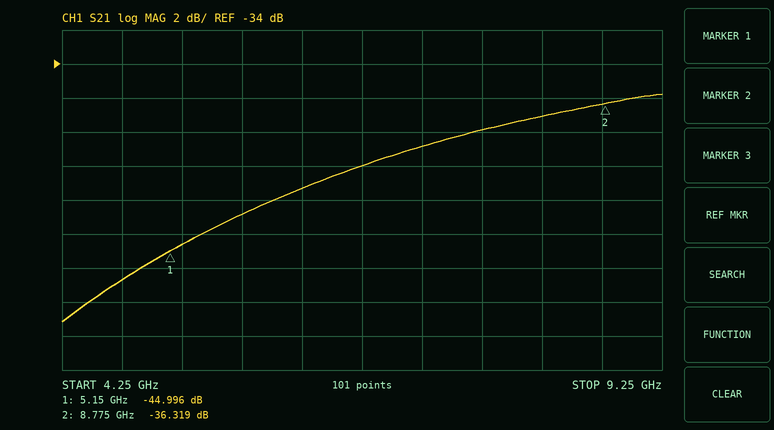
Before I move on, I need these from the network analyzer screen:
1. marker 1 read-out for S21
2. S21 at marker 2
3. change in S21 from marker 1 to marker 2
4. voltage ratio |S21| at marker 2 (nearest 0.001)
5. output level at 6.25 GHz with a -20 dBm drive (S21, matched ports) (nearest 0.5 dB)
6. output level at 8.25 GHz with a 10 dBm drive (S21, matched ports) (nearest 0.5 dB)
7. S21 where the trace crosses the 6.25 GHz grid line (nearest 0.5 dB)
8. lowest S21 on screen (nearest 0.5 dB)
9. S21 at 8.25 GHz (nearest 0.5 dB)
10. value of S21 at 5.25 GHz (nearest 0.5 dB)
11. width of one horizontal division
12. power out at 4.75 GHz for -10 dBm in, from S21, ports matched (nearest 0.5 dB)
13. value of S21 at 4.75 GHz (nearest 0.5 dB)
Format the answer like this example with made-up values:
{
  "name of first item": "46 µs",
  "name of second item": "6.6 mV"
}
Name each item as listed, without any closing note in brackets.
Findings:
{
  "marker 1 read-out for S21": "-44.996 dB",
  "S21 at marker 2": "-36.319 dB",
  "change in S21 from marker 1 to marker 2": "8.677 dB",
  "voltage ratio |S21| at marker 2": "0.015",
  "output level at 6.25 GHz with a -20 dBm drive (S21, matched ports)": "-61.5 dBm",
  "output level at 8.25 GHz with a 10 dBm drive (S21, matched ports)": "-27.0 dBm",
  "S21 where the trace crosses the 6.25 GHz grid line": "-41.5 dB",
  "lowest S21 on screen": "-49.0 dB",
  "S21 at 8.25 GHz": "-37.0 dB",
  "value of S21 at 5.25 GHz": "-44.5 dB",
  "width of one horizontal division": "500 MHz",
  "power out at 4.75 GHz for -10 dBm in, from S21, ports matched": "-56.5 dBm",
  "value of S21 at 4.75 GHz": "-46.5 dB"
}
